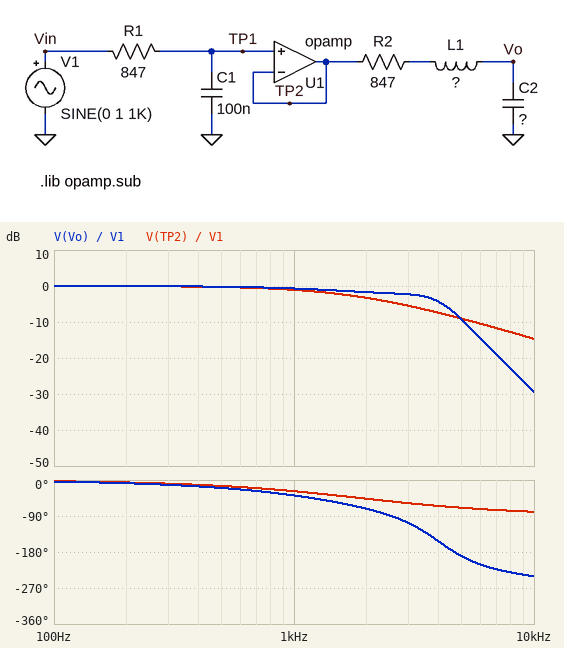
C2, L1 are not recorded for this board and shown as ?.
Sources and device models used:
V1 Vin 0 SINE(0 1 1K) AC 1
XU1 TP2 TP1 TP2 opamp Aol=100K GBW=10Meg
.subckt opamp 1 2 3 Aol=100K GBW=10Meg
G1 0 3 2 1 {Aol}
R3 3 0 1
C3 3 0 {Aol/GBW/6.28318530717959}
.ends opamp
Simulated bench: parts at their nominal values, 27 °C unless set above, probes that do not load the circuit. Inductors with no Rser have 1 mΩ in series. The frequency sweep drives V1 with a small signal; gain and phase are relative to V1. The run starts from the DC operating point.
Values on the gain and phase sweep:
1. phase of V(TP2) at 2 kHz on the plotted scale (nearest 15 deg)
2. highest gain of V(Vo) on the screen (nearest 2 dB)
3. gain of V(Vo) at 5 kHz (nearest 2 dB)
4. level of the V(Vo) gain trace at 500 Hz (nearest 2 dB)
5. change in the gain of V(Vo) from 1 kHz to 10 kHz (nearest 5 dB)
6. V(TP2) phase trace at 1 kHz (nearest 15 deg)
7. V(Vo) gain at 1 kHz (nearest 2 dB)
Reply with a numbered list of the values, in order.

1. -45 deg
2. 0 dB
3. -10 dB
4. 0 dB
5. -30 dB
6. -30 deg
7. 0 dB
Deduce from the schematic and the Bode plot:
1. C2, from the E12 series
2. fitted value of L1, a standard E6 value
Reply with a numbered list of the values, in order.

1. 33 nF
2. 47 mH
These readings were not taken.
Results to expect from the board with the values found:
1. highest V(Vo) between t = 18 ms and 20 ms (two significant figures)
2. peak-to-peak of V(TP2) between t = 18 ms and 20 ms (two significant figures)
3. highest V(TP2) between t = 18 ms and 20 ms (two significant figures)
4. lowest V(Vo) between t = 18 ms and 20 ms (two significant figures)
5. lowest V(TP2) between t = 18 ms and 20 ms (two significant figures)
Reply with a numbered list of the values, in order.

1. 920 mV
2. 1.8 V
3. 880 mV
4. -920 mV
5. -880 mV
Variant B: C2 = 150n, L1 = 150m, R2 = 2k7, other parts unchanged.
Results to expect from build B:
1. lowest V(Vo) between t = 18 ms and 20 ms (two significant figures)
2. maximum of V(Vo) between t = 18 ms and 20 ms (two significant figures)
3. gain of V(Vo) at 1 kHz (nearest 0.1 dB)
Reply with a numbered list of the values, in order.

1. -350 mV
2. 350 mV
3. -9.2 dB
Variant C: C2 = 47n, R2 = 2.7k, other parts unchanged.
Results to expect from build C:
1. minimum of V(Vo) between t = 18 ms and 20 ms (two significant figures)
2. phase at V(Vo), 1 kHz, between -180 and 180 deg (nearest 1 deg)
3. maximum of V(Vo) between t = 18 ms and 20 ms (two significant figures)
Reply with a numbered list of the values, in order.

1. -730 mV
2. -69 deg
3. 730 mV
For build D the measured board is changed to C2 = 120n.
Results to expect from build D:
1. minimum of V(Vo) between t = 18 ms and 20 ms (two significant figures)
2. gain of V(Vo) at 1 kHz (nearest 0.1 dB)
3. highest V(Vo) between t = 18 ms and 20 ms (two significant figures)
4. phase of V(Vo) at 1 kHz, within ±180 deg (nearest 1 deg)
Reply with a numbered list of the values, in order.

1. -880 mV
2. -1.1 dB
3. 880 mV
4. -67 deg
